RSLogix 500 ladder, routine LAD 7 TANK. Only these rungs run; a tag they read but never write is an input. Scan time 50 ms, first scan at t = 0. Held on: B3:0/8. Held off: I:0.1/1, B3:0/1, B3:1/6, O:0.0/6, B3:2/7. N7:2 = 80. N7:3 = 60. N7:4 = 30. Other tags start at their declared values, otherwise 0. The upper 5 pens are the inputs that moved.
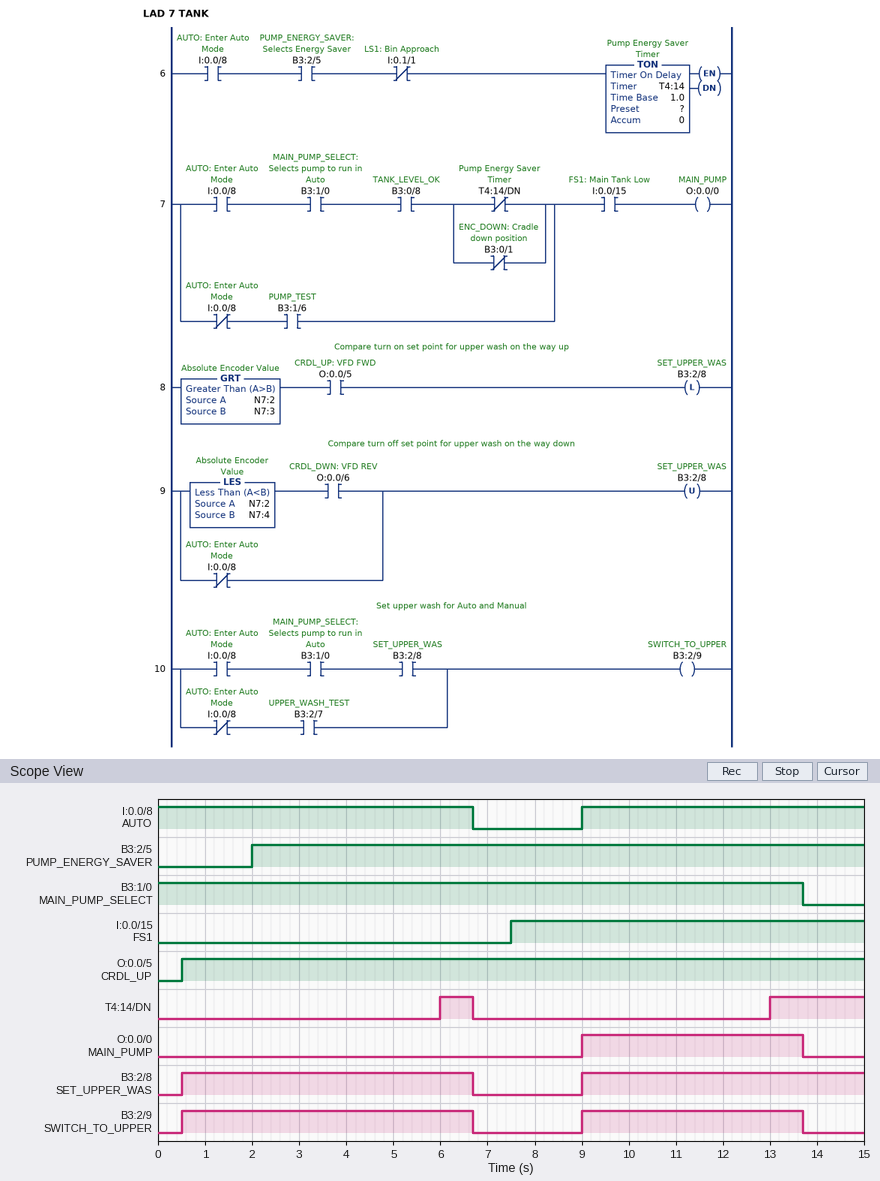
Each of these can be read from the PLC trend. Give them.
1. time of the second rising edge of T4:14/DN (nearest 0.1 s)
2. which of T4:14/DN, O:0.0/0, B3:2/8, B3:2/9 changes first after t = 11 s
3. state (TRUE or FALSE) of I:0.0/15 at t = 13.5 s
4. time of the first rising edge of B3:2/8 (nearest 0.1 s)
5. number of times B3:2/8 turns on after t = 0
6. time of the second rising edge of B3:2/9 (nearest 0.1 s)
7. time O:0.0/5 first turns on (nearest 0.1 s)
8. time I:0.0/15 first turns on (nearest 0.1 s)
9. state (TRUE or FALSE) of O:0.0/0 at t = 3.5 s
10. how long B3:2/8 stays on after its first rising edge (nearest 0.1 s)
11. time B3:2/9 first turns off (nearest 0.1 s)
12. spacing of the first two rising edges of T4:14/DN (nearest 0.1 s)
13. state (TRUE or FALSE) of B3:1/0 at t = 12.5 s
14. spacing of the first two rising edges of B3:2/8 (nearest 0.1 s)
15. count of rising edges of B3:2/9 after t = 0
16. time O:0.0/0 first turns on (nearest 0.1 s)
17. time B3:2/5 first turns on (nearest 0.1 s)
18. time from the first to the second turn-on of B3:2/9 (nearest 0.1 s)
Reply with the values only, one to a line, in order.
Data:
13.0 s
T4:14/DN
TRUE
0.5 s
2
9.0 s
0.5 s
7.5 s
FALSE
6.2 s
6.7 s
7.0 s
TRUE
8.5 s
2
9.0 s
2.0 s
8.5 s
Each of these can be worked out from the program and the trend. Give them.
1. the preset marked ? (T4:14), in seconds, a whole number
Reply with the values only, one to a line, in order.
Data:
4 s
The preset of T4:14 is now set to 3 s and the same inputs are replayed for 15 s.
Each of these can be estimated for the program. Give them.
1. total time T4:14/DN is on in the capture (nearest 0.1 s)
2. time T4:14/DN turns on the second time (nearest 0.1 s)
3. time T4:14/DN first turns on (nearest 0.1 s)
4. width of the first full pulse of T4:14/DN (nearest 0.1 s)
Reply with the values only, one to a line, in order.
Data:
4.7 s
12.0 s
5.0 s
1.7 s
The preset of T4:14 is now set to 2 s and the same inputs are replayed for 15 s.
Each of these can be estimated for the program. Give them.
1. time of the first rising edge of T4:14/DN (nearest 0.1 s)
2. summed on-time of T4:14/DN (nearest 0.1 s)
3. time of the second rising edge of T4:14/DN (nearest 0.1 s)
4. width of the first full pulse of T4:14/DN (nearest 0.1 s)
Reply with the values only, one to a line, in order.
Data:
4.0 s
6.7 s
11.0 s
2.7 s
